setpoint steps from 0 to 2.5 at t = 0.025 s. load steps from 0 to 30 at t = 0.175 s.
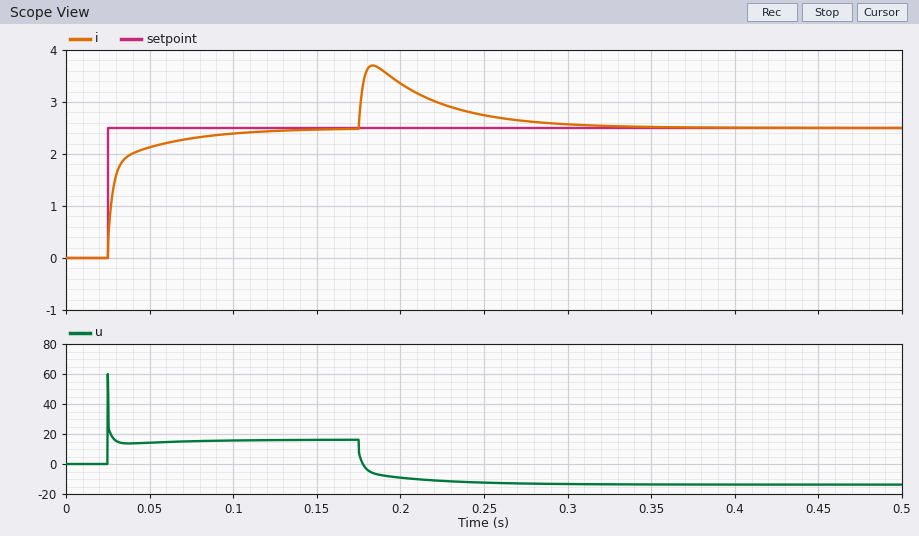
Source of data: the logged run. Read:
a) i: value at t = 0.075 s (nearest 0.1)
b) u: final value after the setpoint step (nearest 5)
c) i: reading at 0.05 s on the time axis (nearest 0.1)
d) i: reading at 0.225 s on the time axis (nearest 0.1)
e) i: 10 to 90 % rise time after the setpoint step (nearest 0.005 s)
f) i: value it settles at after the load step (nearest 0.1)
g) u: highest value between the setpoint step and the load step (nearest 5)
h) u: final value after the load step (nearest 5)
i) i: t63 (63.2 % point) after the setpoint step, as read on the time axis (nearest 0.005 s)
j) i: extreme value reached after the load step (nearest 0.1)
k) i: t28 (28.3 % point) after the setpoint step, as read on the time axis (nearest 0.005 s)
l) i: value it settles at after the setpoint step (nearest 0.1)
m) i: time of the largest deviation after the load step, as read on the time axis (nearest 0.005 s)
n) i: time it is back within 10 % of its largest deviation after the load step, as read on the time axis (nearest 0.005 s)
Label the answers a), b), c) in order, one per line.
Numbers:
a) 2.3
b) 15
c) 2.1
d) 3.0
e) 0.040 s
f) 2.5
g) 60
h) -15
i) 0.030 s
j) 3.7
k) 0.025 s
l) 2.5
m) 0.185 s
n) 0.280 s
